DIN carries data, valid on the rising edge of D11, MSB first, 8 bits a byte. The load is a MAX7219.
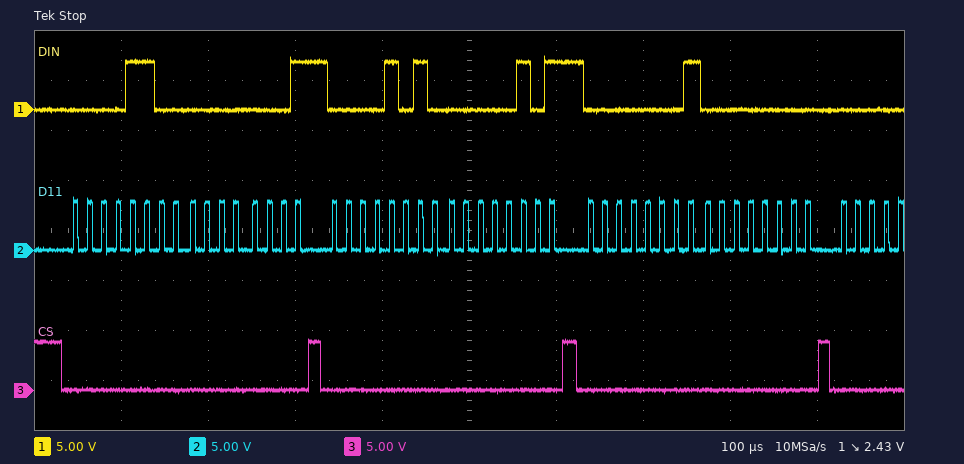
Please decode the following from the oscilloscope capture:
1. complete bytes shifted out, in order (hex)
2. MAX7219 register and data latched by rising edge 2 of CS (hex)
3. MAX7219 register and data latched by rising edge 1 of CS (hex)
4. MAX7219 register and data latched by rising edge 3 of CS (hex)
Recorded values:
0x0C 0x01 0x0A 0x05 0x01 0x00
register 0xA, data 0x05
register 0xC, data 0x01
register 0x1, data 0x00
